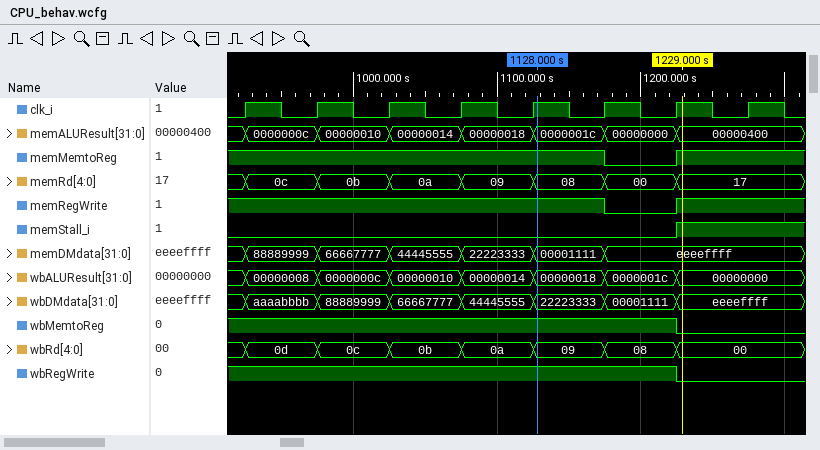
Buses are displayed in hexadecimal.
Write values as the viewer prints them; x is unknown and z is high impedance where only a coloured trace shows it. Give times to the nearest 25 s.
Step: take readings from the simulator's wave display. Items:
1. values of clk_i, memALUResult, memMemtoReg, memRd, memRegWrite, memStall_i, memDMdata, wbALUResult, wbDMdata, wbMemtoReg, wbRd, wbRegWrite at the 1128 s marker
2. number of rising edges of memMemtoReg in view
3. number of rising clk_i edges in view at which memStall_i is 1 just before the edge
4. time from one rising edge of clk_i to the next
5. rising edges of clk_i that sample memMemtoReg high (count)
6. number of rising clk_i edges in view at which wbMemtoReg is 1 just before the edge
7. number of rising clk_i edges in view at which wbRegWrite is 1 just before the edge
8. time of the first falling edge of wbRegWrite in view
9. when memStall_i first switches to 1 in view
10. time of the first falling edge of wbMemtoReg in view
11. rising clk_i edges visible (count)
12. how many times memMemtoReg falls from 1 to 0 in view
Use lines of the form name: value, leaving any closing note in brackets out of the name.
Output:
values of clk_i, memALUResult, memMemtoReg, memRd, memRegWrite, memStall_i, memDMdata, wbALUResult, wbDMdata, wbMemtoReg, wbRd, wbRegWrite at the 1128 s marker: clk_i=1, memALUResult=0000001c, memMemtoReg=1, memRd=08, memRegWrite=1, memStall_i=0, memDMdata=00001111, wbALUResult=00000018, wbDMdata=22223333, wbMemtoReg=1, wbRd=09, wbRegWrite=1
number of rising edges of memMemtoReg in view: 1
number of rising clk_i edges in view at which memStall_i is 1 just before the edge: 1
time from one rising edge of clk_i to the next: 50 s
rising edges of clk_i that sample memMemtoReg high: 7
number of rising clk_i edges in view at which wbMemtoReg is 1 just before the edge: 7
number of rising clk_i edges in view at which wbRegWrite is 1 just before the edge: 7
time of the first falling edge of wbRegWrite in view: 1225 s
when memStall_i first switches to 1 in view: 1225 s
time of the first falling edge of wbMemtoReg in view: 1225 s
rising clk_i edges visible: 8
how many times memMemtoReg falls from 1 to 0 in view: 1
